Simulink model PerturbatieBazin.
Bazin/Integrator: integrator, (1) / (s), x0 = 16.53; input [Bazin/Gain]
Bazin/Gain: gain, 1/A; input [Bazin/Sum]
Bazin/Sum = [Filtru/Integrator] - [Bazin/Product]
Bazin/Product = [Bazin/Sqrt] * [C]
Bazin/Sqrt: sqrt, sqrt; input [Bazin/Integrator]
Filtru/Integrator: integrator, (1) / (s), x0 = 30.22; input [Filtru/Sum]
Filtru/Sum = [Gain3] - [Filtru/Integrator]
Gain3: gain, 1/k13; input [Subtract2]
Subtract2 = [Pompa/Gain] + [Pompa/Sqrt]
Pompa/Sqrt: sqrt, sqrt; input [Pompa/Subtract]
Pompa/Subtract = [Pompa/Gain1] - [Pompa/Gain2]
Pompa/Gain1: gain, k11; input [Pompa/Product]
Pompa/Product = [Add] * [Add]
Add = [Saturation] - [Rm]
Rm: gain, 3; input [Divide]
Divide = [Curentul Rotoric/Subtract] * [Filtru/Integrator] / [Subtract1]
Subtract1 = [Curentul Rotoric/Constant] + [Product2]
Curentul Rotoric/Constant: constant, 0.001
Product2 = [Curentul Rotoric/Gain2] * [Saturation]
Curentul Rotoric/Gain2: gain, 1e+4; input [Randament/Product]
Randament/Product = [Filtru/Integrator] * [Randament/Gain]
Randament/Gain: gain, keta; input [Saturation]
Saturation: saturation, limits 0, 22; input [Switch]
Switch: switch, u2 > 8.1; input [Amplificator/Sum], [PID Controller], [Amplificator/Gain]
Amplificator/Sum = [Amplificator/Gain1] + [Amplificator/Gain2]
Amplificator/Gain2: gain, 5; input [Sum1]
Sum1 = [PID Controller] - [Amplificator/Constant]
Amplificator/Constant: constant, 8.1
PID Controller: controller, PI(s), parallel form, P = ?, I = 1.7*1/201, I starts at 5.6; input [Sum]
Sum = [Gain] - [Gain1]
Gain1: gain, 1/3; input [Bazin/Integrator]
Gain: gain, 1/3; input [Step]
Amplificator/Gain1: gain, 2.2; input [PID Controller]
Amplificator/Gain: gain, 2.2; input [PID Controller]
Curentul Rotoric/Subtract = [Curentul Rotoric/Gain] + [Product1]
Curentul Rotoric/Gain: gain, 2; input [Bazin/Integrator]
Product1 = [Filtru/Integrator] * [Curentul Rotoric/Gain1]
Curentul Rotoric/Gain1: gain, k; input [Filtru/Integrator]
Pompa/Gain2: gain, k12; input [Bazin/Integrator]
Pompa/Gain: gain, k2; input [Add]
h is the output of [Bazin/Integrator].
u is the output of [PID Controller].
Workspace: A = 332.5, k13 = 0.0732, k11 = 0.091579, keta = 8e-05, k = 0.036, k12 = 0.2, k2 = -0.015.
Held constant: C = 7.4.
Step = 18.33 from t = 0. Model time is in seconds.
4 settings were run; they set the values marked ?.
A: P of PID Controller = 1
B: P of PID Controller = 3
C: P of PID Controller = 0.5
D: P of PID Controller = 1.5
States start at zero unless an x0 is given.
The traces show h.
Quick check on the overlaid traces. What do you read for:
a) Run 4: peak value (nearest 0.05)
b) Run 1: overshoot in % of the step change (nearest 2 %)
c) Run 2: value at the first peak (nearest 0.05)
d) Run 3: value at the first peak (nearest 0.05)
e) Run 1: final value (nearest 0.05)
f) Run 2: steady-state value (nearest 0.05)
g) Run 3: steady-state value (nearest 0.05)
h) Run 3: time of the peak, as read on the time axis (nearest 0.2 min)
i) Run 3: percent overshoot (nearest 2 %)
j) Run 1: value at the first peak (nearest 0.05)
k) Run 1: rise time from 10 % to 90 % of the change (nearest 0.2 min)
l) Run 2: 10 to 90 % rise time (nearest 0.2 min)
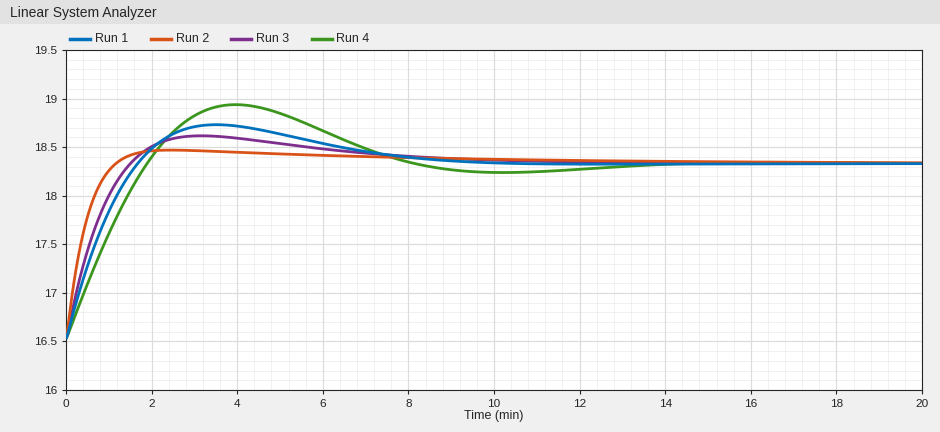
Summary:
18.95
22 %
18.45
18.60
18.35
18.35
18.35
3.2 min
16 %
18.75
1.2 min
0.8 min
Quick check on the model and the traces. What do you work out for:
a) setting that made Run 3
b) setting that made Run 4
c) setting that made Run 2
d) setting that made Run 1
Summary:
D
C
B
A
